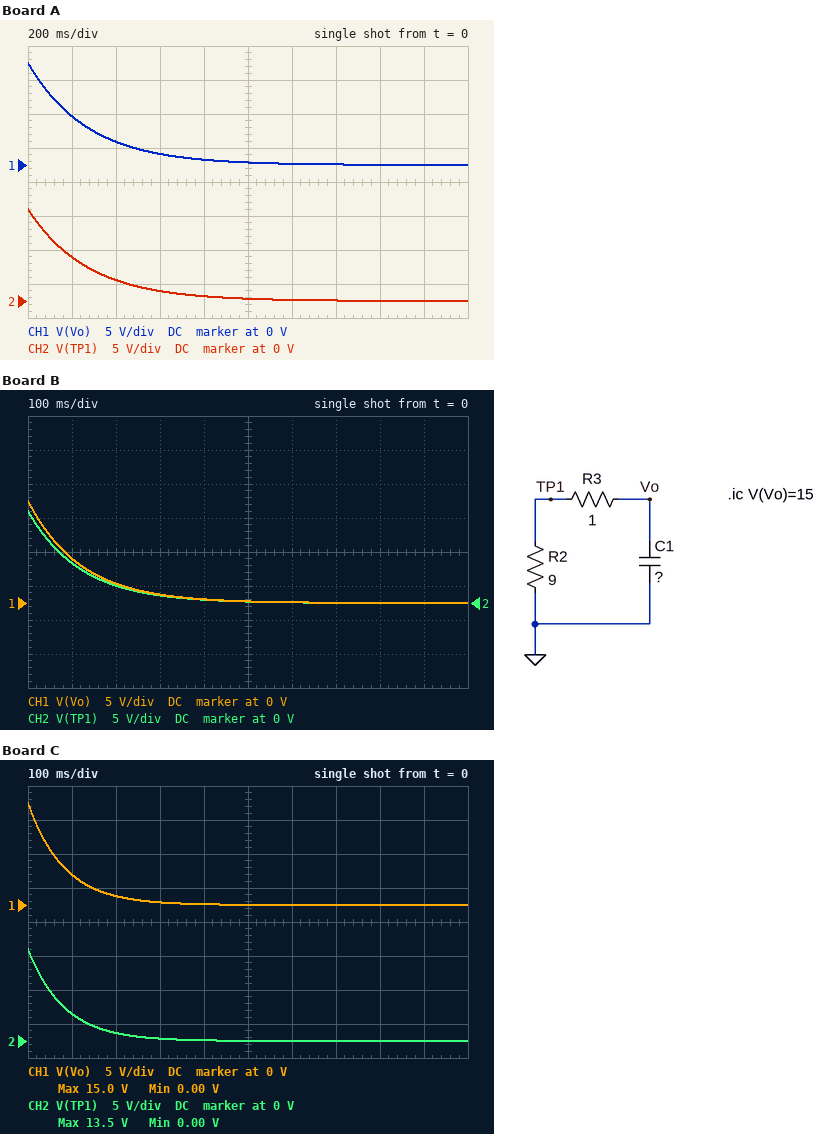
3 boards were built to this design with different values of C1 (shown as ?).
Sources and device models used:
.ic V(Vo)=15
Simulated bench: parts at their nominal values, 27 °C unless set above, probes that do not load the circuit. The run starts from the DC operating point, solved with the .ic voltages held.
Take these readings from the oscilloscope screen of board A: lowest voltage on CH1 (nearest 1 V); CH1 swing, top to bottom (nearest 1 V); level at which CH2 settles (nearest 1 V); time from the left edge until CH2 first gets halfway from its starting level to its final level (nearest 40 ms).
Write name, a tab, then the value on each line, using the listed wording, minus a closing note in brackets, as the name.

lowest voltage on CH1	0 V
CH1 swing, top to bottom	15 V
level at which CH2 settles	0 V
time from the left edge until CH2 first gets halfway from its starting level to its final level	200 ms
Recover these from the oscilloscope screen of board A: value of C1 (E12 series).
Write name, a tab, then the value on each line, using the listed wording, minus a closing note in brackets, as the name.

value of C1	27 mF
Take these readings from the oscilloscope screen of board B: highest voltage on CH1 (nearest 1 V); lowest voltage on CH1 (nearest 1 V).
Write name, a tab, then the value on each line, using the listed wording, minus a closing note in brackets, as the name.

highest voltage on CH1	15 V
lowest voltage on CH1	0 V
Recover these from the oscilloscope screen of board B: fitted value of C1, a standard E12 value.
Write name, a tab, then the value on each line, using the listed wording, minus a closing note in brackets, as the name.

fitted value of C1, a standard E12 value	12 mF
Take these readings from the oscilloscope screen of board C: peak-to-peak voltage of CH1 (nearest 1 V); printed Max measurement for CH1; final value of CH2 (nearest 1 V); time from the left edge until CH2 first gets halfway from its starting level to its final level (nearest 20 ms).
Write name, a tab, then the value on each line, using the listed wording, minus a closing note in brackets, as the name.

peak-to-peak voltage of CH1	15 V
printed Max measurement for CH1	15.0 V
final value of CH2	0 V
time from the left edge until CH2 first gets halfway from its starting level to its final level	60 ms
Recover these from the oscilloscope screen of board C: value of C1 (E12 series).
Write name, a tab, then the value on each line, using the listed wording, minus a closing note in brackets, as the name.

value of C1	8.2 mF
